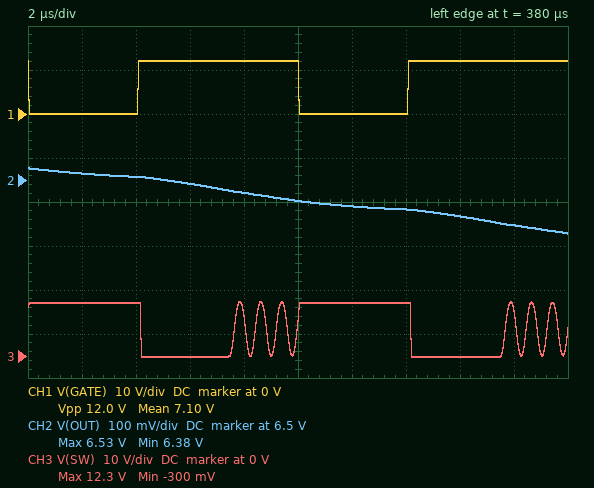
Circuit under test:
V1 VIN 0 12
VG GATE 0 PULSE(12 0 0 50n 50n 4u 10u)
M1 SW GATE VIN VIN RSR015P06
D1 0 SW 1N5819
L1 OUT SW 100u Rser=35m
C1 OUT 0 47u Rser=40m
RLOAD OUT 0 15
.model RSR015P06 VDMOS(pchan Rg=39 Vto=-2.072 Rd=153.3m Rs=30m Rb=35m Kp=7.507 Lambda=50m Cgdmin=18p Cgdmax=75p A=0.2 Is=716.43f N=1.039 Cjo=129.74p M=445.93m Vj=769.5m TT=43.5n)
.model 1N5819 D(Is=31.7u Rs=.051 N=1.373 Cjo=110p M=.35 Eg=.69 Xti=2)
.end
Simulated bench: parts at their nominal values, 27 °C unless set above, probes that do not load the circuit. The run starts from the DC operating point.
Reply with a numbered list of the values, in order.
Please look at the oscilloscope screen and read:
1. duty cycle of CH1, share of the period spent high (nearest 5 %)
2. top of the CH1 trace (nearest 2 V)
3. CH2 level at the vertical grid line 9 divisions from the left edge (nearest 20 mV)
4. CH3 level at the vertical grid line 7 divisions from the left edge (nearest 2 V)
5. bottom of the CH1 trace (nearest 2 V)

1. 60 %
2. 12 V
3. 6.40 V
4. 12 V
5. 0 V
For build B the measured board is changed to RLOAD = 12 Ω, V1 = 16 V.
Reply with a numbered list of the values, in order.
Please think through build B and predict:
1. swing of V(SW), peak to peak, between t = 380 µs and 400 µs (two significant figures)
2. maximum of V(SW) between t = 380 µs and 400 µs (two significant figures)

1. 84 mV
2. 16 V
